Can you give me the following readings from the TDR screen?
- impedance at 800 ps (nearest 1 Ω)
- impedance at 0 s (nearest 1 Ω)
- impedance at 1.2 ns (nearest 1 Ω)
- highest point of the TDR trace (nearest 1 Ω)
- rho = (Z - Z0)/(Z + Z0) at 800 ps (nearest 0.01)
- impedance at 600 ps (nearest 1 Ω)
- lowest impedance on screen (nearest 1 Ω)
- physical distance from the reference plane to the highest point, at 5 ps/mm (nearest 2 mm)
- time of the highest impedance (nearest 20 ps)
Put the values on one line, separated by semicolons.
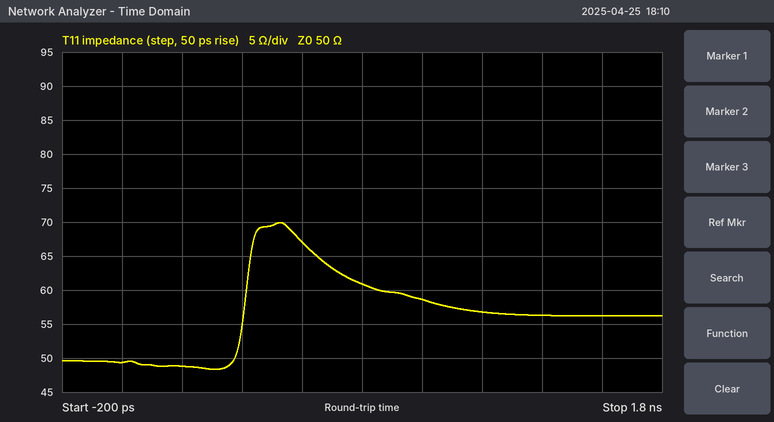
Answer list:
61 Ω; 49 Ω; 57 Ω; 70 Ω; +0.10; 67 Ω; 48 Ω; 52 mm; 520 ps
